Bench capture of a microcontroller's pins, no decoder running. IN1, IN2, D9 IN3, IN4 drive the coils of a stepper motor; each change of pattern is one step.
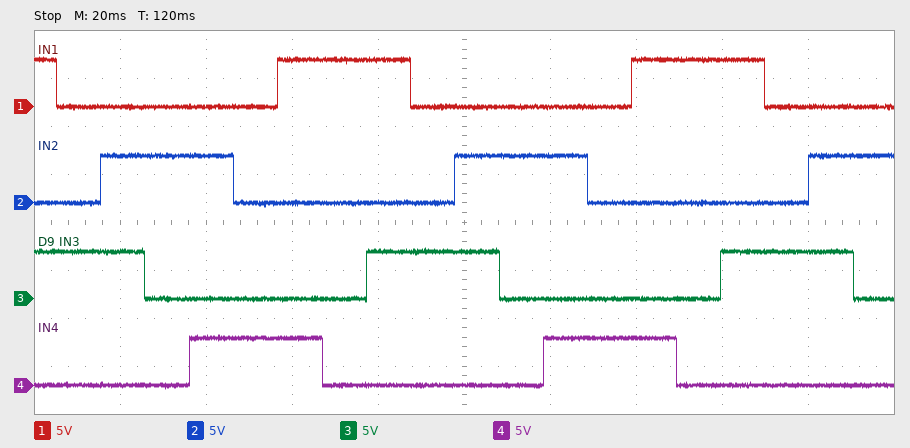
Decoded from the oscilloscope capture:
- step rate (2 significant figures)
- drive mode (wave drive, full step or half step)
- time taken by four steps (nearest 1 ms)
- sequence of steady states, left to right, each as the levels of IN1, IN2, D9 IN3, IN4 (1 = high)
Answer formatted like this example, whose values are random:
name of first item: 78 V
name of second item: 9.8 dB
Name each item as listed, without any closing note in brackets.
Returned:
step rate: 97 steps/s
drive mode: half step
time taken by four steps: 41 ms
sequence of steady states, left to right, each as the levels of IN1, IN2, D9 IN3, IN4: 1010 0010 0110 0100 0101 0001 1001 1000 1010 0010 0110 0100 0101 0001 1001 1000 1010 0010 0110 0100
